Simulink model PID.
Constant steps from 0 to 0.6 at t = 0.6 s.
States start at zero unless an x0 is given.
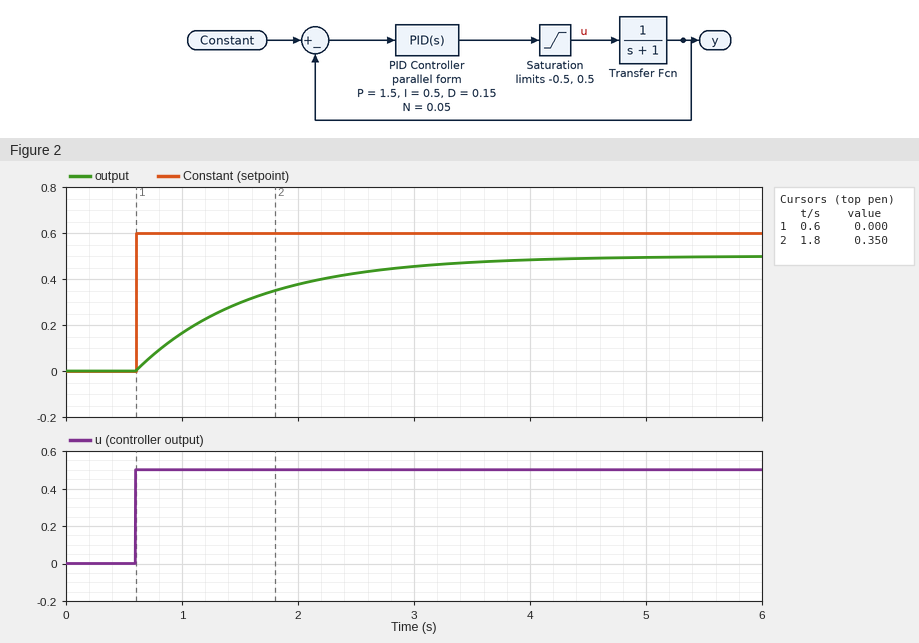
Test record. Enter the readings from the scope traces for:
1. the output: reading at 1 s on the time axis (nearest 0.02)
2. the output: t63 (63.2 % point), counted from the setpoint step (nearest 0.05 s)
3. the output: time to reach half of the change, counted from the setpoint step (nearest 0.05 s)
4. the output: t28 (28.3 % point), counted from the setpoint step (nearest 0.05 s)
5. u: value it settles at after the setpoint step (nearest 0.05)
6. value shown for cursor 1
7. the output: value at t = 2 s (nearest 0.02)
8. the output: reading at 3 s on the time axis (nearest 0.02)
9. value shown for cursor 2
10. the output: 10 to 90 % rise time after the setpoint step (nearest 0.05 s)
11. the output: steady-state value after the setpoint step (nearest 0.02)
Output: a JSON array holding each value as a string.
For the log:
["0.16", "1.00 s", "0.70 s", "0.35 s", "0.50", "0.000", "0.38", "0.46", "0.350", "2.20 s", "0.50"]
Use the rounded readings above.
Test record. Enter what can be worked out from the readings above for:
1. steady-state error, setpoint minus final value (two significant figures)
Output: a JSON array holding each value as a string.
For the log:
["0.10"]
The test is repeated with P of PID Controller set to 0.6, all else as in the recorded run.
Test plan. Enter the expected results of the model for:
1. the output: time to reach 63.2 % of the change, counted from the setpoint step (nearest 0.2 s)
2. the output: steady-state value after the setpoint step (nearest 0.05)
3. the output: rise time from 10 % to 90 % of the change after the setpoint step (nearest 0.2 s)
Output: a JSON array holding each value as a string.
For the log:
["1.4 s", "0.50", "2.6 s"]
